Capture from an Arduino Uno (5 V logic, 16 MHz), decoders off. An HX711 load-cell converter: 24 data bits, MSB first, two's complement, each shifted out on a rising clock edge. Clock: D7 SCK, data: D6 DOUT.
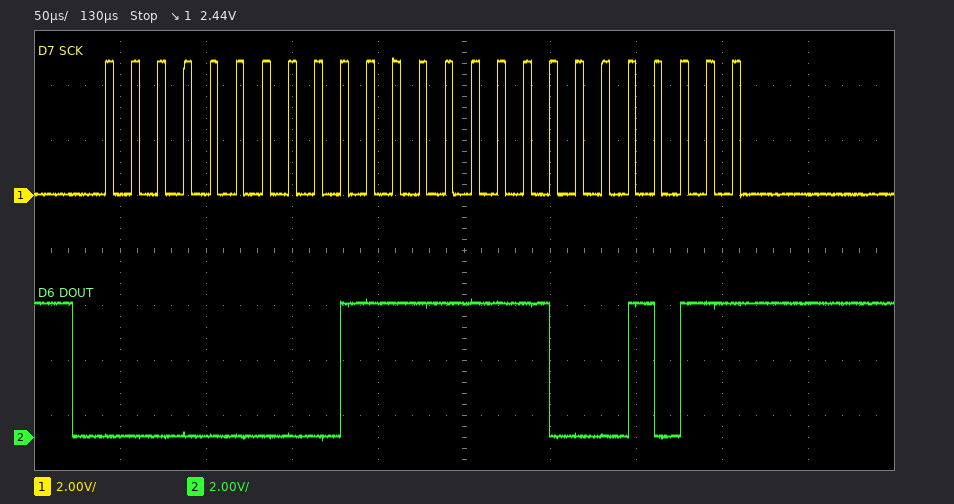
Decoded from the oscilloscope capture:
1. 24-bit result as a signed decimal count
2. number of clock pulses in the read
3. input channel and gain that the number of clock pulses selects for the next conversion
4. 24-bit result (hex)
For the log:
32651
25
channel A, gain 128
0x007F8B
